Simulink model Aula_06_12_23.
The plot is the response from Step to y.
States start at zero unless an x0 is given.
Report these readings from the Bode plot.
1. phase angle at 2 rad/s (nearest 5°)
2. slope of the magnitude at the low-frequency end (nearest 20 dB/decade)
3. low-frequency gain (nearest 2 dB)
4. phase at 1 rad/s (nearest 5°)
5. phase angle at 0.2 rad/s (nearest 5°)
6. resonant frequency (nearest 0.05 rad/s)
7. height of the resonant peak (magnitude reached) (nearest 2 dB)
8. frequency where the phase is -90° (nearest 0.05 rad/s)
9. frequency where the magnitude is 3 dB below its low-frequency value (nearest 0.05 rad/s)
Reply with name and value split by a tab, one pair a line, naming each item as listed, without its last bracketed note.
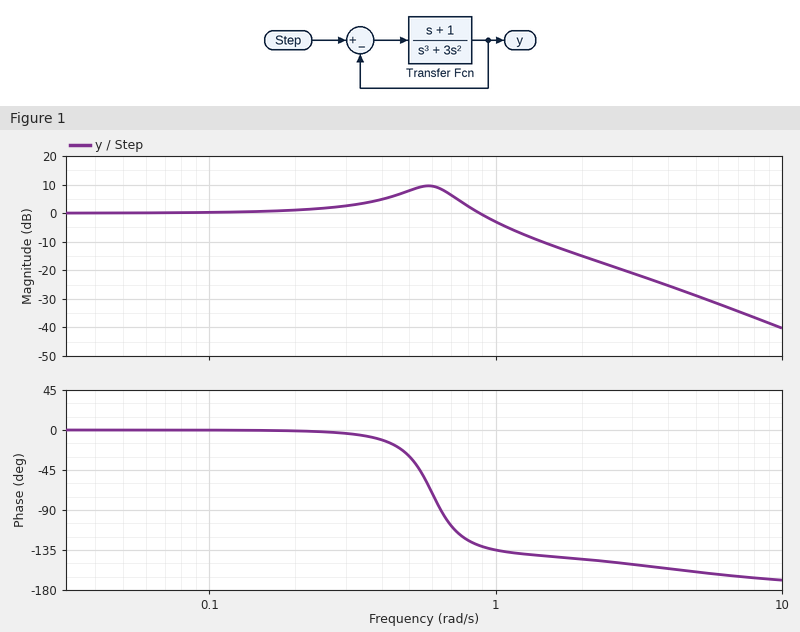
phase angle at 2 rad/s	-145°
slope of the magnitude at the low-frequency end	0 dB/decade
low-frequency gain	0 dB
phase at 1 rad/s	-135°
phase angle at 0.2 rad/s	0°
resonant frequency	0.60 rad/s
height of the resonant peak (magnitude reached)	10 dB
frequency where the phase is -90°	0.65 rad/s
frequency where the magnitude is 3 dB below its low-frequency value	1.00 rad/s
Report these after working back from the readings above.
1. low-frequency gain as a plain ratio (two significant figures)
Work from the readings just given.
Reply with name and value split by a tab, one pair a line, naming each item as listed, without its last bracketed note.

low-frequency gain as a plain ratio	1.0
